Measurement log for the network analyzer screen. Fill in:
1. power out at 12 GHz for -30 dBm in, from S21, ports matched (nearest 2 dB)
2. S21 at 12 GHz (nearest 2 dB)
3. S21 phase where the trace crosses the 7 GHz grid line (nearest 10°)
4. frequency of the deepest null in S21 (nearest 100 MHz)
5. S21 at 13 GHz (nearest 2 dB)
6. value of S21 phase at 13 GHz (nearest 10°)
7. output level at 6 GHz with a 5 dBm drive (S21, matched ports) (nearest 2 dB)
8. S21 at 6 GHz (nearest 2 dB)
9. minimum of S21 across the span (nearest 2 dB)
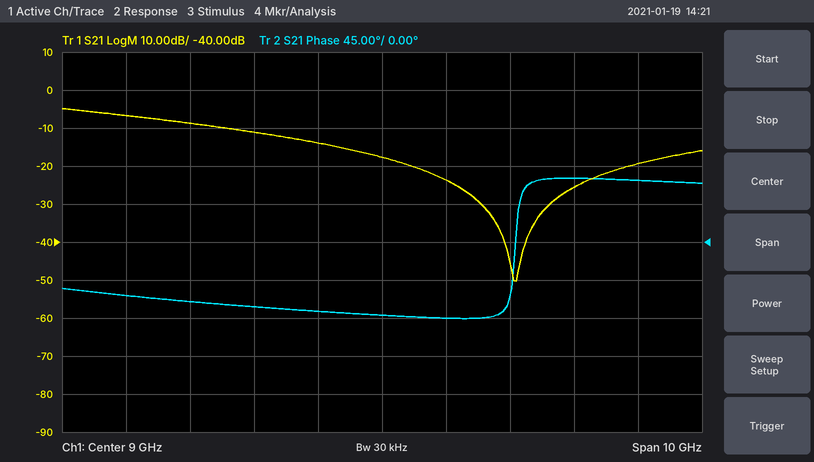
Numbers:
-56 dBm
-26 dB
-80°
11.1 GHz
-20 dB
70°
-4 dBm
-8 dB
-50 dB
